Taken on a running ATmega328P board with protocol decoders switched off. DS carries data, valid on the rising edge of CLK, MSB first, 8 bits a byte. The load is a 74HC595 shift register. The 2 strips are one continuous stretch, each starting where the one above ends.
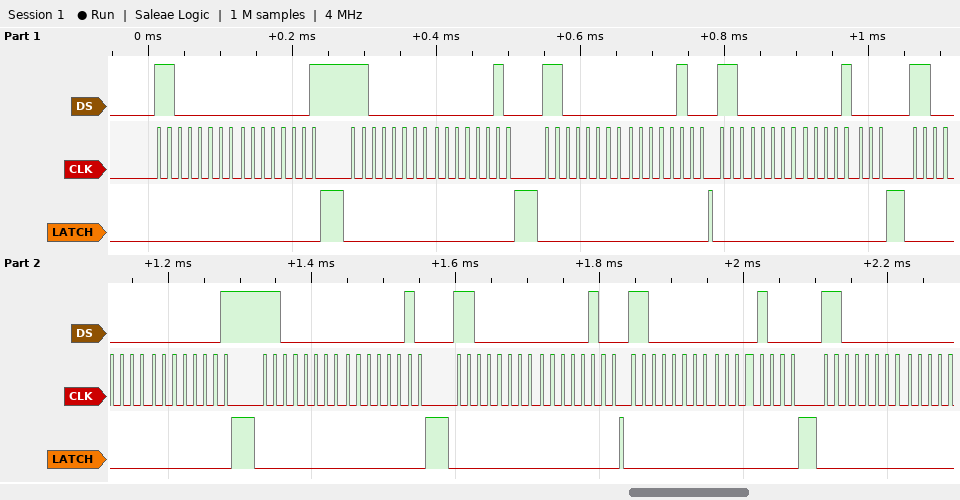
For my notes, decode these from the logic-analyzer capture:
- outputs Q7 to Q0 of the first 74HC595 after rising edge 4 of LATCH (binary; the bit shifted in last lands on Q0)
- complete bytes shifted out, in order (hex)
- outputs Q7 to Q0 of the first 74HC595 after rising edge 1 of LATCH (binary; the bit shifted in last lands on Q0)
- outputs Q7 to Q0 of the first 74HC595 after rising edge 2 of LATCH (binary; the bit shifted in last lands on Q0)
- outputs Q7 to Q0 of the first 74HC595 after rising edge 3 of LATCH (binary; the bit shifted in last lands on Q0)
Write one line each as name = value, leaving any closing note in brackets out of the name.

outputs Q7 to Q0 of the first 74HC595 after rising edge 4 of LATCH = 00001000
complete bytes shifted out, in order = C0 01 C0 02 C0 04 C0 08 C0 01 C0 02 C0 04 C0 08 C0
outputs Q7 to Q0 of the first 74HC595 after rising edge 1 of LATCH = 00000001
outputs Q7 to Q0 of the first 74HC595 after rising edge 2 of LATCH = 00000010
outputs Q7 to Q0 of the first 74HC595 after rising edge 3 of LATCH = 00000100
